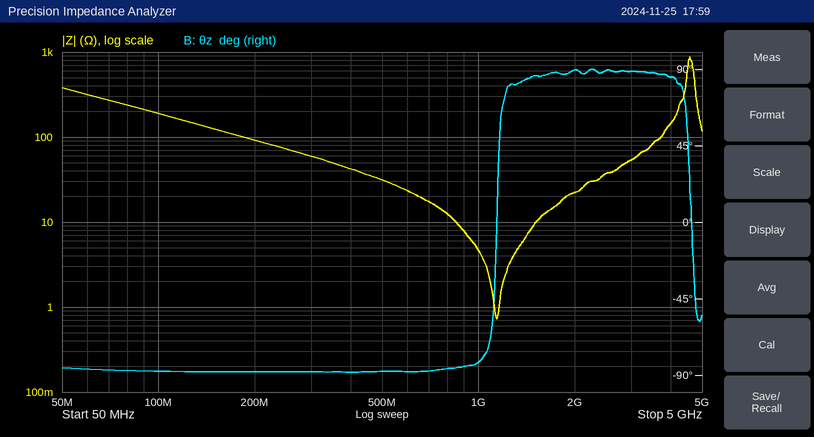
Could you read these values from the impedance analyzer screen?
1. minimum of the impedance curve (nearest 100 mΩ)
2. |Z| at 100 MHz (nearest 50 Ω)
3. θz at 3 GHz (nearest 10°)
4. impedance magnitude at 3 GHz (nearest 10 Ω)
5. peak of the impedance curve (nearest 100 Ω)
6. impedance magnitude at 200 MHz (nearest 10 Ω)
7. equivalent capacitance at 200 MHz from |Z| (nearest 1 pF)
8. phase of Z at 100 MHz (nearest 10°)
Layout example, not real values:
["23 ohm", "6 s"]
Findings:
["700 mΩ", "200 Ω", "90°", "50 Ω", "900 Ω", "90 Ω", "9 pF", "-90°"]
